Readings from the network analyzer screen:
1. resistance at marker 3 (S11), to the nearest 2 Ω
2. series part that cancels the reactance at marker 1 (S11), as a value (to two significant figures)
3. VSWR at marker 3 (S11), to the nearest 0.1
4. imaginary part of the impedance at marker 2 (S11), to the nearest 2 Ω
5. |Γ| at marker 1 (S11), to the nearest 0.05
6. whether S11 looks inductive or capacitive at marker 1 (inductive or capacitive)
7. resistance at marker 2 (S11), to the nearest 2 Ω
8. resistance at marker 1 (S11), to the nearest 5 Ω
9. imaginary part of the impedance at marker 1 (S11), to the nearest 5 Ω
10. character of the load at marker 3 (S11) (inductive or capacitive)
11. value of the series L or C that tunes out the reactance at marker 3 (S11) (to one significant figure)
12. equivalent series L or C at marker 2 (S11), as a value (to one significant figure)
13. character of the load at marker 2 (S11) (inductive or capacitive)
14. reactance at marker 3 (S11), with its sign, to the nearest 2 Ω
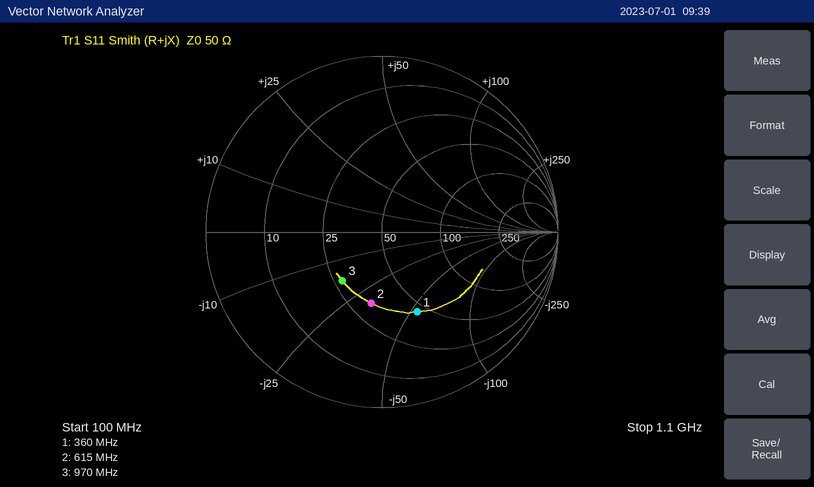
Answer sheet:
28 Ω
24 nH
2.1
-32 Ω
0.50
capacitive
32 Ω
45 Ω
-55 Ω
capacitive
3 nH
8 pF
capacitive
-18 Ω
